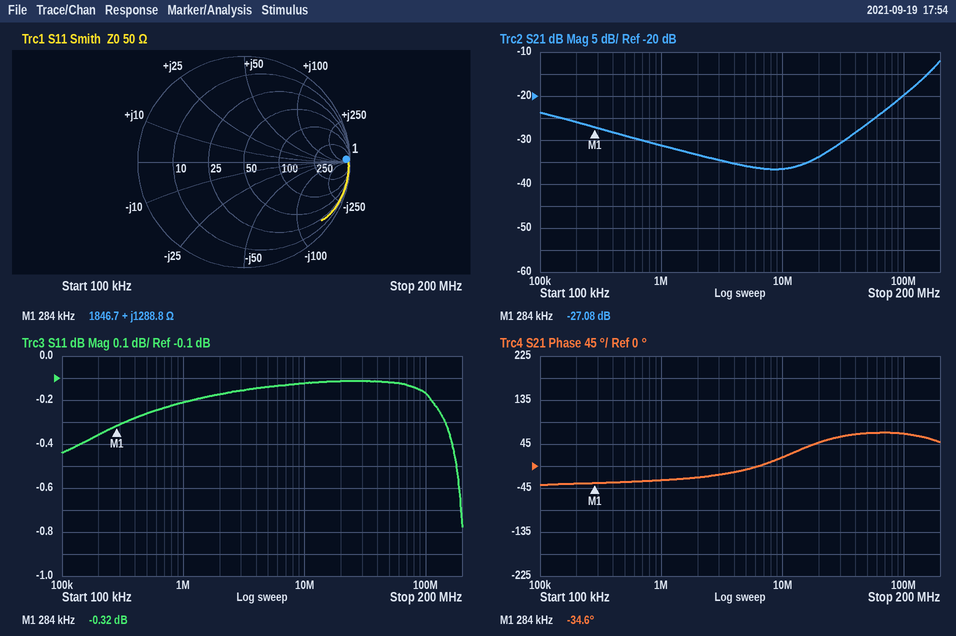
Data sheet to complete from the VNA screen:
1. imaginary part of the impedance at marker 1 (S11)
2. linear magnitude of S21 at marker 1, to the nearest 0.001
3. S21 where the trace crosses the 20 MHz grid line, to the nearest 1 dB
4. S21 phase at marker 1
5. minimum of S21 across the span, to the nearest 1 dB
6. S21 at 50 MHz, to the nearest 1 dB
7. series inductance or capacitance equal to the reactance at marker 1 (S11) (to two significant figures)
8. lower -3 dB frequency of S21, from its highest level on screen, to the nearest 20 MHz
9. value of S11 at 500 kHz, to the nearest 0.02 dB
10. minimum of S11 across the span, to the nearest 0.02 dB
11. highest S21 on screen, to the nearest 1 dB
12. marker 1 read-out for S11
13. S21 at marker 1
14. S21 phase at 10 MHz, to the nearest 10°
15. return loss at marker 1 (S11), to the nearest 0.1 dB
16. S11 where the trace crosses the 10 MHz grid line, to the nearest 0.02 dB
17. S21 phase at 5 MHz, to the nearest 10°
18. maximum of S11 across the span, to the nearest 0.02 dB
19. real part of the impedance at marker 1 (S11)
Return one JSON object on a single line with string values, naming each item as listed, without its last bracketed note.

{"imaginary part of the impedance at marker 1": "+1288.8 Ω", "linear magnitude of S21 at marker 1, to the nearest 0.001": "0.044", "S21 where the trace crosses the 20 MHz grid line, to the nearest 1 dB": "-34 dB", "S21 phase at marker 1": "-34.6°", "minimum of S21 across the span, to the nearest 1 dB": "-37 dB", "S21 at 50 MHz, to the nearest 1 dB": "-26 dB", "series inductance or capacitance equal to the reactance at marker 1 (S11)": "720 µH", "lower -3 dB frequency of S21, from its highest level on screen, to the nearest 20 MHz": "160 MHz", "value of S11 at 500 kHz, to the nearest 0.02 dB": "-0.26 dB", "minimum of S11 across the span, to the nearest 0.02 dB": "-0.78 dB", "highest S21 on screen, to the nearest 1 dB": "-12 dB", "marker 1 read-out for S11": "-0.32 dB", "S21 at marker 1": "-27.08 dB", "S21 phase at 10 MHz, to the nearest 10°": "20°", "return loss at marker 1 (S11), to the nearest 0.1 dB": "0.3 dB", "S11 where the trace crosses the 10 MHz grid line, to the nearest 0.02 dB": "-0.12 dB", "S21 phase at 5 MHz, to the nearest 10°": "-10°", "maximum of S11 across the span, to the nearest 0.02 dB": "-0.12 dB", "real part of the impedance at marker 1": "1846.7 Ω"}
